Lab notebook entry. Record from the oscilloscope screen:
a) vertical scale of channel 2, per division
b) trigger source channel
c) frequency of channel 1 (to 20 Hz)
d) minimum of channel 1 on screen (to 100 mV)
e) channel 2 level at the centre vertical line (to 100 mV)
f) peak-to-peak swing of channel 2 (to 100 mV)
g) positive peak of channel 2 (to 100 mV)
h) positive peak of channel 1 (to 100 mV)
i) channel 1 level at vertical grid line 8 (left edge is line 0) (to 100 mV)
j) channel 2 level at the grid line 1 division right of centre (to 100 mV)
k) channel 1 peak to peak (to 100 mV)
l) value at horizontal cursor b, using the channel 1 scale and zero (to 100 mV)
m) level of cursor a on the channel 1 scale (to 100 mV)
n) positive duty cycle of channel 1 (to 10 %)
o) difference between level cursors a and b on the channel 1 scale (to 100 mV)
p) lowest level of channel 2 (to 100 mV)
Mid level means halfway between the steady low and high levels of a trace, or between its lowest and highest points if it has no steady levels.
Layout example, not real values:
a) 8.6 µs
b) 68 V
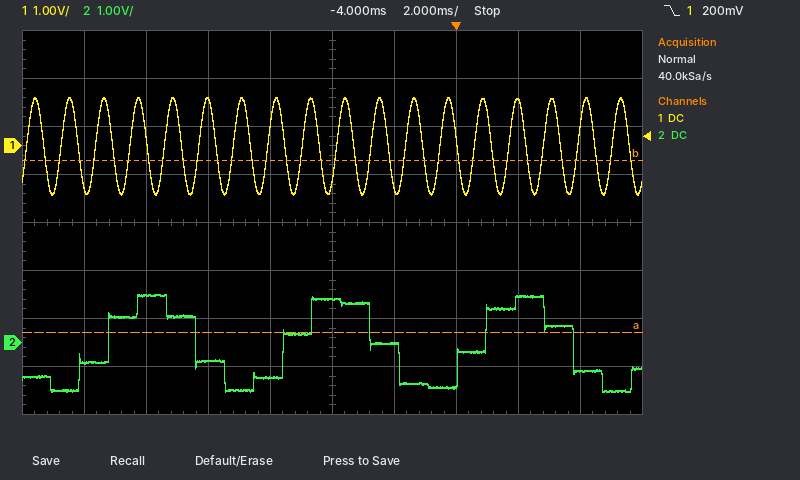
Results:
a) 1 V
b) channel 1
c) 900 Hz
d) -1.0 V
e) 900 mV
f) 2.0 V
g) 1.0 V
h) 1.0 V
i) 900 mV
j) 0.0 V
k) 2.0 V
l) -300 mV
m) -3.9 V
n) 50 %
o) 3.6 V
p) -1.0 V
